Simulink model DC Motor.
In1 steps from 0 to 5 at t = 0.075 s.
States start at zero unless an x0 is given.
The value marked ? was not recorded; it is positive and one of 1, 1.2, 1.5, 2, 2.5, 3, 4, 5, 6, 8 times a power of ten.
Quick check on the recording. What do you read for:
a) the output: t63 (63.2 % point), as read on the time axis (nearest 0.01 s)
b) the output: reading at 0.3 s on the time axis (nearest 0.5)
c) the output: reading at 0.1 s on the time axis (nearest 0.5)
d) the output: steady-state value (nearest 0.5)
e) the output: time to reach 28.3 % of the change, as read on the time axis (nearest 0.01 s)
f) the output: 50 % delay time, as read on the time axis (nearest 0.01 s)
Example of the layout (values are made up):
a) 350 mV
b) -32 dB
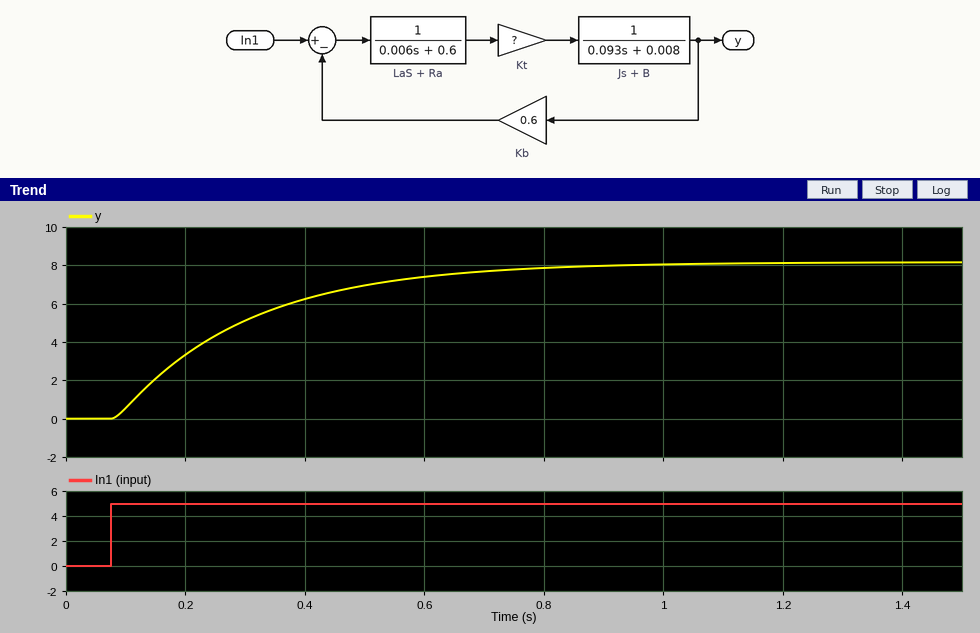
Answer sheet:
a) 0.30 s
b) 5.0
c) 0.5
d) 8.0
e) 0.16 s
f) 0.24 s
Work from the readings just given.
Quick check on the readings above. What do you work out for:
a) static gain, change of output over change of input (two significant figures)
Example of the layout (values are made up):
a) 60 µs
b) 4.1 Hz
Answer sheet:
a) 1.6
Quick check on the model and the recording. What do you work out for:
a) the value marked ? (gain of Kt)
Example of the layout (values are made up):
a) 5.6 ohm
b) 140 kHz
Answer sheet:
a) 0.4
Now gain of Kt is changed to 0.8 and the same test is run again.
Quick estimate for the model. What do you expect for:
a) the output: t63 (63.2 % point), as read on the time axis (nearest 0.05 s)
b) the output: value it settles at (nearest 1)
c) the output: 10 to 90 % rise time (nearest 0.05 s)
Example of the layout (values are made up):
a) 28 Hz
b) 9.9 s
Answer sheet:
a) 0.20 s
b) 8
c) 0.25 s
